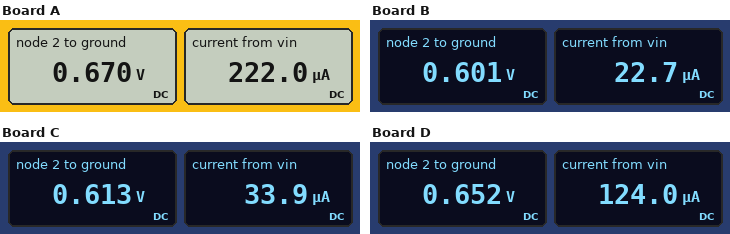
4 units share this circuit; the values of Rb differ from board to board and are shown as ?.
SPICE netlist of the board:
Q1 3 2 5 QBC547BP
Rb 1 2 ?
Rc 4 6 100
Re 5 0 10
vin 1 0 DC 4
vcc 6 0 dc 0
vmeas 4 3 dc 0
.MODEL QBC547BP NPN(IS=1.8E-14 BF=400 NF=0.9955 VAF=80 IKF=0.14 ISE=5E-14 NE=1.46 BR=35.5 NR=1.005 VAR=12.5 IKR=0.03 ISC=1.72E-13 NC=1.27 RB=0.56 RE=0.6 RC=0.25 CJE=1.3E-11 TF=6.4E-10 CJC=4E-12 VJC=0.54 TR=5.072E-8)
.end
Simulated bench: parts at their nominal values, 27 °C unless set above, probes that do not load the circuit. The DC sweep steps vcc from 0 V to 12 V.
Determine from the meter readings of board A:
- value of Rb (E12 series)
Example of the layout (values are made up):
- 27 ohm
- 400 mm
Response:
- 15 kΩ
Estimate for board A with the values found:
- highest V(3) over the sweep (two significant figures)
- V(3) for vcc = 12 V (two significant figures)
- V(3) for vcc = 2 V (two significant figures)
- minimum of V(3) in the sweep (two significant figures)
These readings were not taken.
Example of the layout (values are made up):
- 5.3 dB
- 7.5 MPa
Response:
- 7.1 V
- 7.1 V
- 250 mV
- -1.6 mV
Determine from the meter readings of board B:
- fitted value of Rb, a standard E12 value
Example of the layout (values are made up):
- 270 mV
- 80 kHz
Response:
- 150 kΩ
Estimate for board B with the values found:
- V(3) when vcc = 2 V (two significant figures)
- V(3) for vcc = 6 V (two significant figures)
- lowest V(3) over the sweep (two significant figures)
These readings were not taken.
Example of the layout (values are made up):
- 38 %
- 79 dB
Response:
- 1.4 V
- 5.3 V
- -1.2 mV
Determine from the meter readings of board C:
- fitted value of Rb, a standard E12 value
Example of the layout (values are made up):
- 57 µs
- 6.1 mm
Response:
- 100 kΩ
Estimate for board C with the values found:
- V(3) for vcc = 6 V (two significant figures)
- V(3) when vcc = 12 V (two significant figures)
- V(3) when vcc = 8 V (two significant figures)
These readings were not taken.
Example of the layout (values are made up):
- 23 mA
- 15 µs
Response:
- 5.0 V
- 11 V
- 7.0 V
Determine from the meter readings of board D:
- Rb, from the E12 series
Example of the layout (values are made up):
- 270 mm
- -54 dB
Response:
- 27 kΩ
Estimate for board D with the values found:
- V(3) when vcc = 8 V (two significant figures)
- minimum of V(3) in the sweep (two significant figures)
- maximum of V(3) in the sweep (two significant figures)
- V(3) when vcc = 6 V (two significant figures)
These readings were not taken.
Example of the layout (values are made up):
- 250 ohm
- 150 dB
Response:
- 4.9 V
- -2.1 mV
- 8.8 V
- 3.0 V
